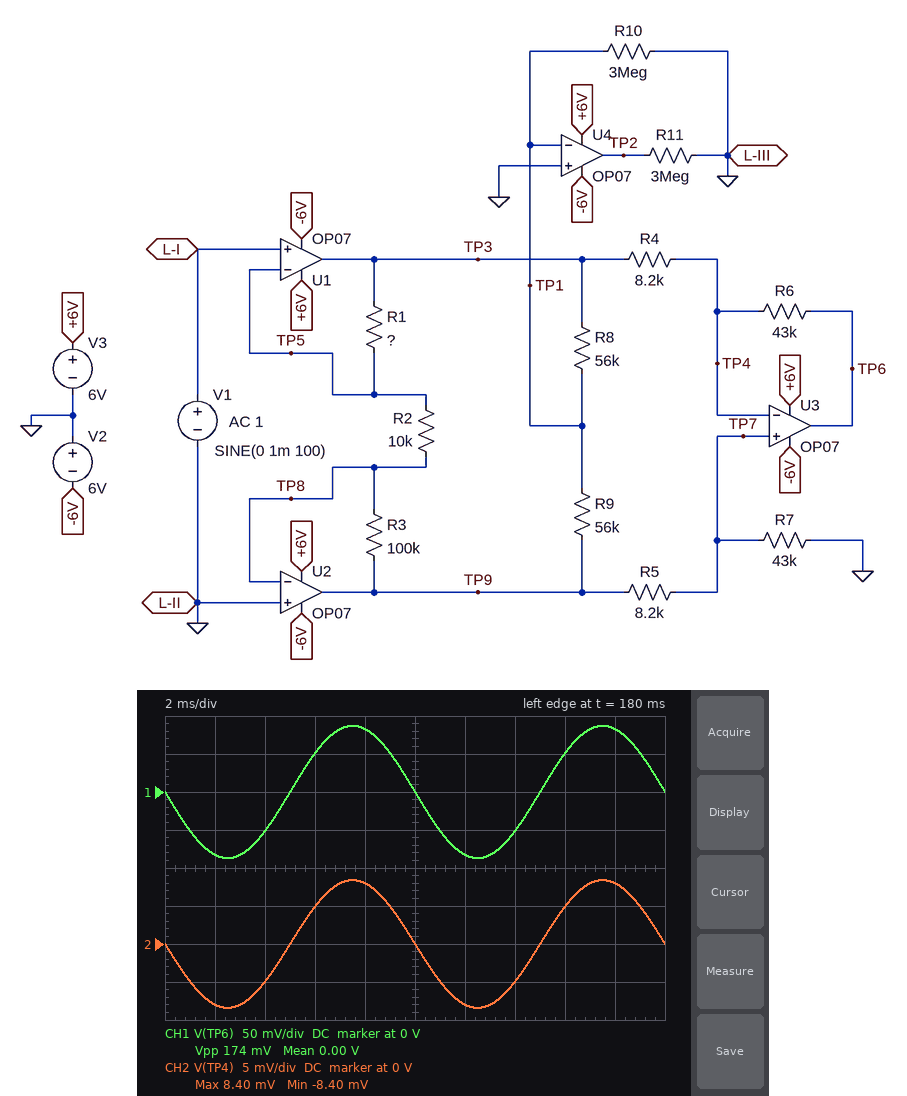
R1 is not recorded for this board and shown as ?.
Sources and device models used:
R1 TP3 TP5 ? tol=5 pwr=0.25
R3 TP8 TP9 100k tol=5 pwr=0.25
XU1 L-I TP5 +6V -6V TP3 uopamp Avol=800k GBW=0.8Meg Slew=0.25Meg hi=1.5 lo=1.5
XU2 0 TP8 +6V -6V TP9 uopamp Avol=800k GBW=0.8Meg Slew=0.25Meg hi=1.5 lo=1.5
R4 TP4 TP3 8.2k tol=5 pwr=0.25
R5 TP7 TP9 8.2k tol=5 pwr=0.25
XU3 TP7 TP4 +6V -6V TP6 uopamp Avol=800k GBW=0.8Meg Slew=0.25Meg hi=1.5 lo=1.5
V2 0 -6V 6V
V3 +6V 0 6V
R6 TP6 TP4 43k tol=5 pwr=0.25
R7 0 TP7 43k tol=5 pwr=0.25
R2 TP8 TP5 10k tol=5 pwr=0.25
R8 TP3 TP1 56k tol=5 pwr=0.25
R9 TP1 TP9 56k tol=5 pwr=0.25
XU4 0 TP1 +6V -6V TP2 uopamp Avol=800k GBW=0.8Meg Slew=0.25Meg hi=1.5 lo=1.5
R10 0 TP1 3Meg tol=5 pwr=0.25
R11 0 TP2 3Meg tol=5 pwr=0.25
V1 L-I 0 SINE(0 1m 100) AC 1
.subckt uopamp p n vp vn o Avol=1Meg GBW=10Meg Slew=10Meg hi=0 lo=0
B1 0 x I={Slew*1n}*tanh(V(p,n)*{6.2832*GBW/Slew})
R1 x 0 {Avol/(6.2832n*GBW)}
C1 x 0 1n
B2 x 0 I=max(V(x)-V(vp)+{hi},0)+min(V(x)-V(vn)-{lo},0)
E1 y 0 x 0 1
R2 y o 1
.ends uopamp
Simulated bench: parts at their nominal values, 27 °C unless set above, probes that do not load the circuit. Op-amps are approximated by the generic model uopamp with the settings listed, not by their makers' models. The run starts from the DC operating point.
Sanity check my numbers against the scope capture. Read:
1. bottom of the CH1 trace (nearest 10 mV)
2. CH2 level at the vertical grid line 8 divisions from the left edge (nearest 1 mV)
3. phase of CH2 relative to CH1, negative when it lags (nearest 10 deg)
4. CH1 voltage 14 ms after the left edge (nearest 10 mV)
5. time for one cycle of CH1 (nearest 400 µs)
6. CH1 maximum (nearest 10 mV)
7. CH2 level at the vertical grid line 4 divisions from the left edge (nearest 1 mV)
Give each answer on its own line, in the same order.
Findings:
-90 mV
5 mV
0 deg
-50 mV
10.0 ms
90 mV
8 mV
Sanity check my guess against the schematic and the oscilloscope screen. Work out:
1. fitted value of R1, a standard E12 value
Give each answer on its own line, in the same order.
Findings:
56 kΩ
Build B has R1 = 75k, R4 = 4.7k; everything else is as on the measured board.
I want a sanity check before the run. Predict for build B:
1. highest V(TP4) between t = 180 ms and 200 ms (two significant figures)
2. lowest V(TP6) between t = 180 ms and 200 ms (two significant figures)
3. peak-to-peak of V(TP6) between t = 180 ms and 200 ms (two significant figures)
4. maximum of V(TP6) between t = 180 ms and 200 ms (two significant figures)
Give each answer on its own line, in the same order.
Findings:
8.4 mV
-160 mV
330 mV
160 mV
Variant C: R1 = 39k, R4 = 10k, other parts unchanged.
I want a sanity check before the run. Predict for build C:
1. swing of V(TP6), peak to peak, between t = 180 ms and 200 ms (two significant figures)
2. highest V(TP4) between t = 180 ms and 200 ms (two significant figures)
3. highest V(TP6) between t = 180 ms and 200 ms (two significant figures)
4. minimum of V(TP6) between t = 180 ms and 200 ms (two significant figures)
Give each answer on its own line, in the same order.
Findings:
130 mV
8.4 mV
66 mV
-66 mV
